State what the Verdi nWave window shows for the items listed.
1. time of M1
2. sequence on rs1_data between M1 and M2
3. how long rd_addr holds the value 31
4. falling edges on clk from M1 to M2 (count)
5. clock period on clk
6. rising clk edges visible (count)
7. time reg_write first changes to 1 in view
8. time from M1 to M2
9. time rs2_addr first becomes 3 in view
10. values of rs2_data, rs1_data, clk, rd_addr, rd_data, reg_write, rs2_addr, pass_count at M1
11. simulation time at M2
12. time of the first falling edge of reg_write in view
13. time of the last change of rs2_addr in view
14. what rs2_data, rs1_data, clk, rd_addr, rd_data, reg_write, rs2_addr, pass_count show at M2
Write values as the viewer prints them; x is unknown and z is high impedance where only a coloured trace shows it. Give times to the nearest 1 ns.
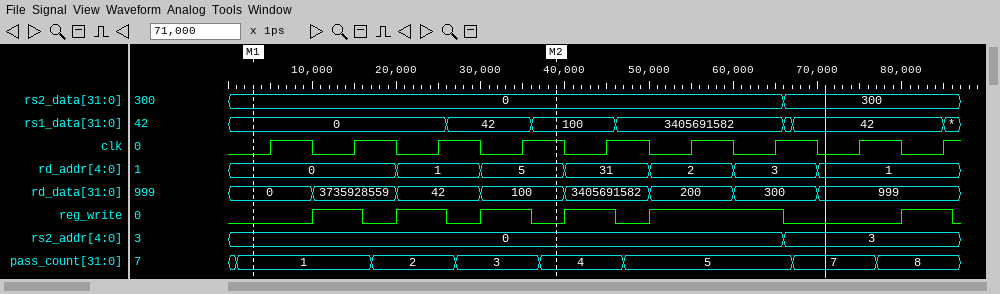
3 ns
0, 42, 100
10 ns
3
10 ns
9
10 ns
36 ns
66 ns
rs2_data=0, rs1_data=0, clk=0, rd_addr=0, rd_data=0, reg_write=0, rs2_addr=0, pass_count=1
39 ns
16 ns
66 ns
rs2_data=0, rs1_data=100, clk=1, rd_addr=5, rd_data=100, reg_write=0, rs2_addr=0, pass_count=4
